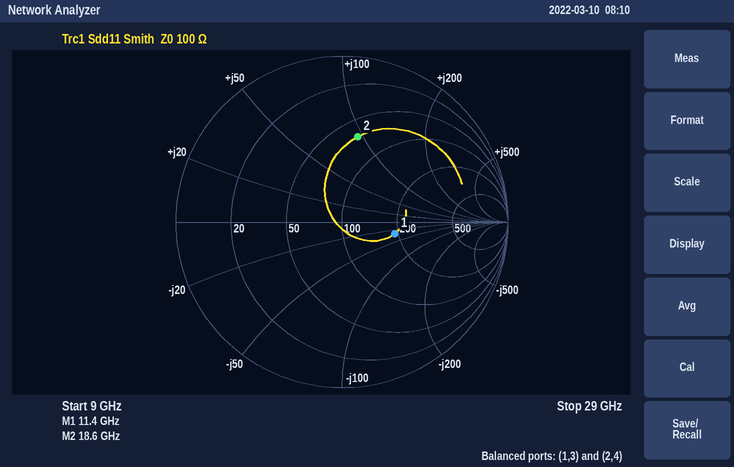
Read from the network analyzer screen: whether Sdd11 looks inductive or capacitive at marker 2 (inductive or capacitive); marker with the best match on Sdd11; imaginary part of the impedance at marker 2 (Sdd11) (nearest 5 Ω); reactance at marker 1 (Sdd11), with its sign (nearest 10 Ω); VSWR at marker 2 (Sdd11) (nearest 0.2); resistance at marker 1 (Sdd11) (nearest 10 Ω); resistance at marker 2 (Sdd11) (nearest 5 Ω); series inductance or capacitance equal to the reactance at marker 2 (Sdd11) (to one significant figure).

inductive
marker 1
+95 Ω
-30 Ω
3.2
190 Ω
65 Ω
800 pH
